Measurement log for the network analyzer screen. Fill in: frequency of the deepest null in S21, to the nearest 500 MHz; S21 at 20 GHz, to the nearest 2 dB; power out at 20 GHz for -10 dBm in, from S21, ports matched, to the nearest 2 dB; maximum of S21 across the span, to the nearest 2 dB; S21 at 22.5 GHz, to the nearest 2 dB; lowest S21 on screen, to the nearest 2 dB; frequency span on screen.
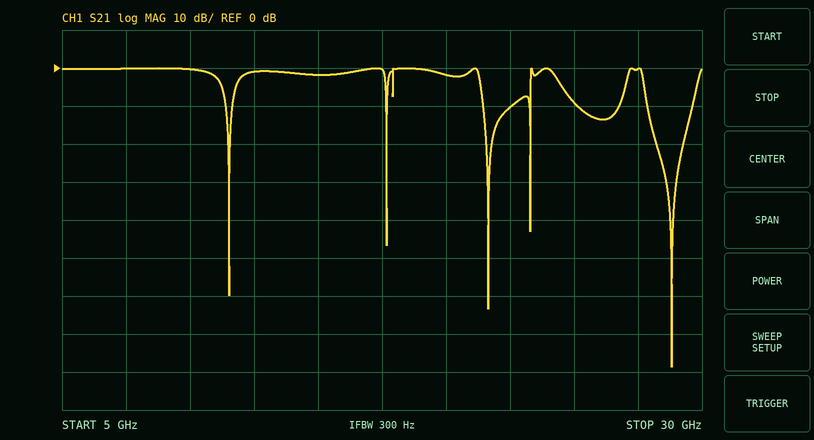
29.0 GHz
-2 dB
-12 dBm
0 dB
-10 dB
-78 dB
25 GHz
